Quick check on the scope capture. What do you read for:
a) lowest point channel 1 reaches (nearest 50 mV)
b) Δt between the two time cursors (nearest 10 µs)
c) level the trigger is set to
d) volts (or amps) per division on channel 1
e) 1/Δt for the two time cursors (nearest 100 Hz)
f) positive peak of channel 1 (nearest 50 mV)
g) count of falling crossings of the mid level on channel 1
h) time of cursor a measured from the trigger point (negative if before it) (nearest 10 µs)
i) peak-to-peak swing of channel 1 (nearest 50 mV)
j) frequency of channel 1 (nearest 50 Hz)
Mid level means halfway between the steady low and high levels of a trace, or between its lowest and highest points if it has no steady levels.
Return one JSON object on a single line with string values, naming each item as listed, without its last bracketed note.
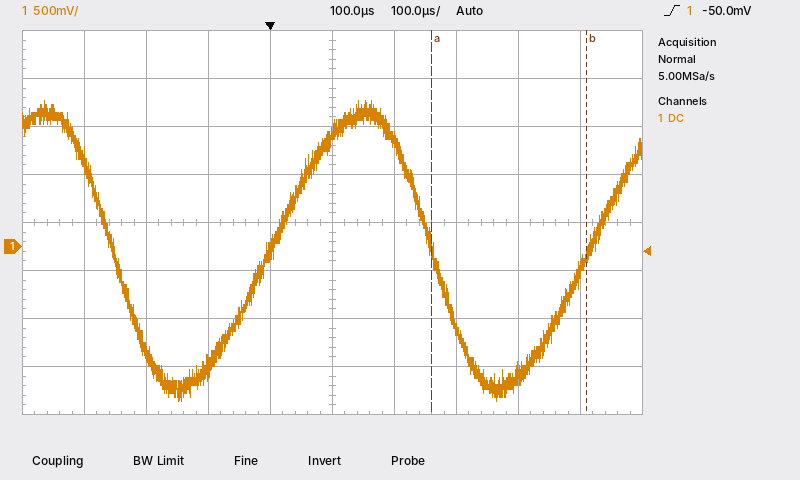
{"lowest point channel 1 reaches": "-1.60 V", "Δt between the two time cursors": "250 µs", "level the trigger is set to": "-50.0 mV", "volts (or amps) per division on channel 1": "500 mV", "1/Δt for the two time cursors": "4.0 kHz", "positive peak of channel 1": "1.50 V", "count of falling crossings of the mid level on channel 1": "2", "time of cursor a measured from the trigger point (negative if before it)": "+260 µs", "peak-to-peak swing of channel 1": "3.10 V", "frequency of channel 1": "1.95 kHz"}
